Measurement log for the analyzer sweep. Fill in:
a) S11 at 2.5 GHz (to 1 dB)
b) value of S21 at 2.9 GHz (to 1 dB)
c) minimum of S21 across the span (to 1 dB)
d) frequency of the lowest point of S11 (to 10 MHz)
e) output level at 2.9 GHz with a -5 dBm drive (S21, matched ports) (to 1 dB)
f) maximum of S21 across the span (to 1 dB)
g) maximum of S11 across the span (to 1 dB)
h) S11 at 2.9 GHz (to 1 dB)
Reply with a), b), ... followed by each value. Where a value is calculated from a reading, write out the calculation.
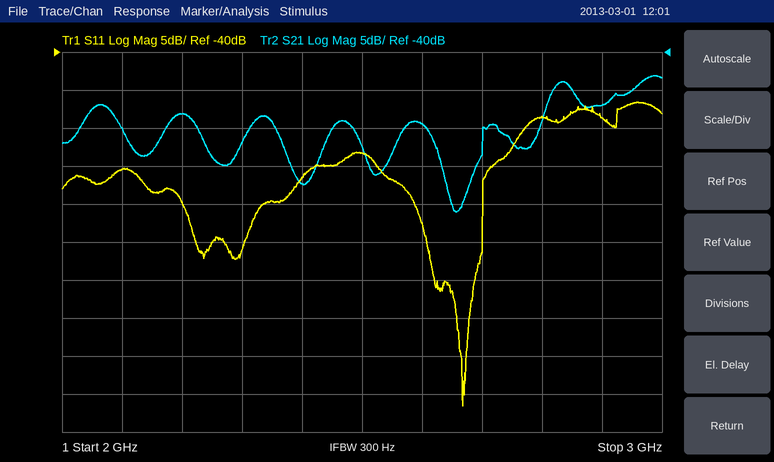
a) -53 dB
b) -47 dB
c) -61 dB
d) 2.67 GHz
e) -5 dBm + (-47 dB) = -52 dBm
f) -43 dB
g) -47 dB
h) -49 dB
